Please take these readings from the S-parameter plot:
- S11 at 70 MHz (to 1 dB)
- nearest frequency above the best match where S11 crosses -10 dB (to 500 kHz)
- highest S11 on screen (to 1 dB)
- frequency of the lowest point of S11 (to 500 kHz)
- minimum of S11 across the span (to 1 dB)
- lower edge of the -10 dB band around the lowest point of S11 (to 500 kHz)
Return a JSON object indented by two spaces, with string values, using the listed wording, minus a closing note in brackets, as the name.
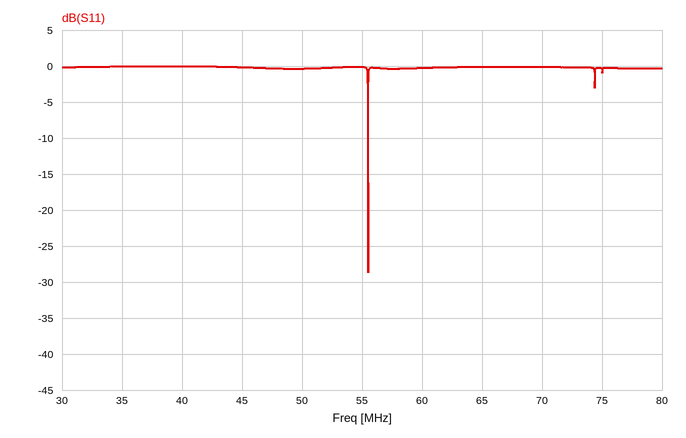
{
  "S11 at 70 MHz": "0 dB",
  "nearest frequency above the best match where S11 crosses -10 dB": "55.5 MHz",
  "highest S11 on screen": "0 dB",
  "frequency of the lowest point of S11": "55.5 MHz",
  "minimum of S11 across the span": "-29 dB",
  "lower edge of the -10 dB band around the lowest point of S11": "55.5 MHz"
}
